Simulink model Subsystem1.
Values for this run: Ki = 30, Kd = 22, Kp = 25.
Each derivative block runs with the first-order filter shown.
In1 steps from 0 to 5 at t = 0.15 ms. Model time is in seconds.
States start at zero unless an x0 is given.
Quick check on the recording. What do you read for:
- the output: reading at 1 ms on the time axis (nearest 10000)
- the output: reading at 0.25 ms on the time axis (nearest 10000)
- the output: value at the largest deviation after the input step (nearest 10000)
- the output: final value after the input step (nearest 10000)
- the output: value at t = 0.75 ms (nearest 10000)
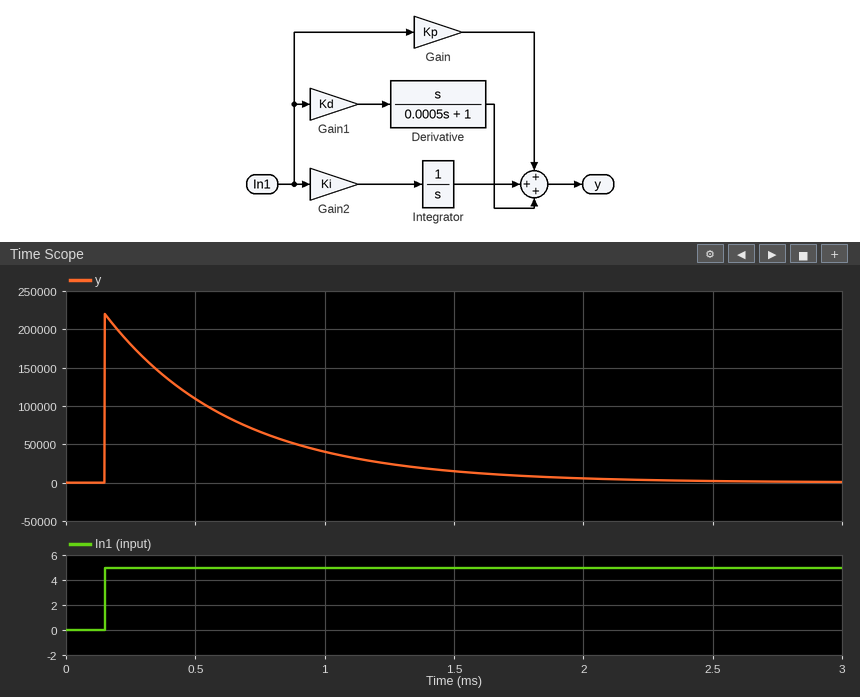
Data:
40000
180000
220000
0
70000
